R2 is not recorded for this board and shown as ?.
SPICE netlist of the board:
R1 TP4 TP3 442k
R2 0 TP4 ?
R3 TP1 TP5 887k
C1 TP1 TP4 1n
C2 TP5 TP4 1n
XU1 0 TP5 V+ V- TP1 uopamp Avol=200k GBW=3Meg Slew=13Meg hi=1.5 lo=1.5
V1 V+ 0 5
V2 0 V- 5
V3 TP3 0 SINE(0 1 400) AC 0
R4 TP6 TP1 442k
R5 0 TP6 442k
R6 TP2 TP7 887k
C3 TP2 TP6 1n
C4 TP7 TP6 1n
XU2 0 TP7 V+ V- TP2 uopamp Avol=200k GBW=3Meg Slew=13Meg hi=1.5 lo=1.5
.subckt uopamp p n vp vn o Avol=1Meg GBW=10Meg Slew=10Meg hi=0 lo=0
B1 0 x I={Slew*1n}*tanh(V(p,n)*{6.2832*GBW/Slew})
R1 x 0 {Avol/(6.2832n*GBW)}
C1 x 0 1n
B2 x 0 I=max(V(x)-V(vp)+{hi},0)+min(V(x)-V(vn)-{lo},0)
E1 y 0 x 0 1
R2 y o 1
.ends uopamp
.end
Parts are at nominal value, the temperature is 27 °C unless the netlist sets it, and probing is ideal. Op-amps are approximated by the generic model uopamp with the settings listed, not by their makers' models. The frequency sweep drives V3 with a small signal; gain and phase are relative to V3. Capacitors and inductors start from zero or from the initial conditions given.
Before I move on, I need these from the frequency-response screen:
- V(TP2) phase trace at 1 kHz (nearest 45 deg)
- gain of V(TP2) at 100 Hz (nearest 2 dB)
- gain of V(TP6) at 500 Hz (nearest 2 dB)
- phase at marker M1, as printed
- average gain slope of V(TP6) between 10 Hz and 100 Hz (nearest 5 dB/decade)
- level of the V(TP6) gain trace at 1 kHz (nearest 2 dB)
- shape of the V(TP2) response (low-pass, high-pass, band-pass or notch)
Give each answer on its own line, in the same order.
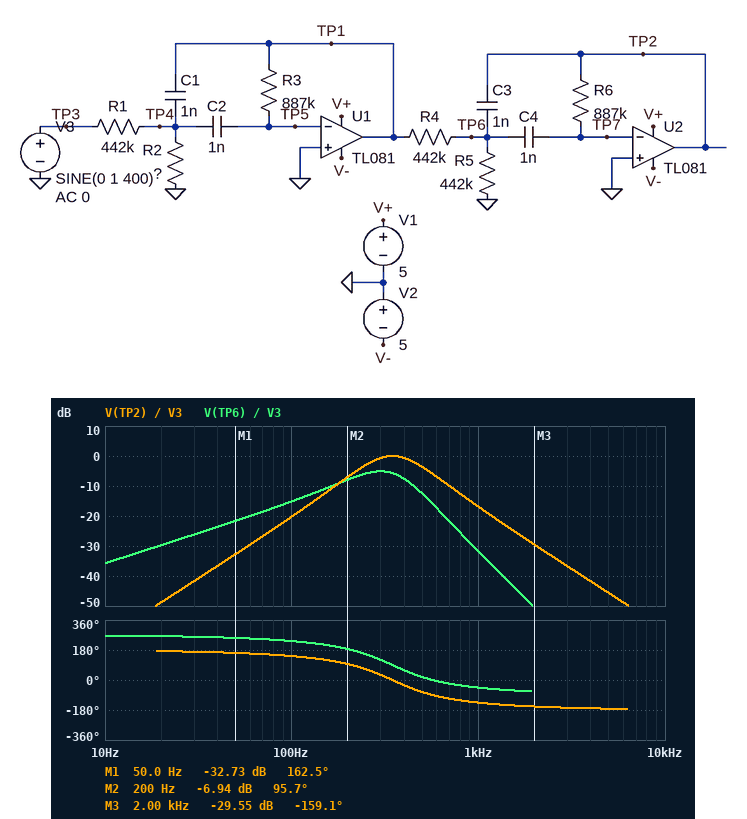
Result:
-135 deg
-20 dB
-12 dB
162.5 deg
20 dB/decade
-32 dB
band-pass
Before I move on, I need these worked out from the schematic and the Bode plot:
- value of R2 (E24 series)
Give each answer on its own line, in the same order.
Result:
620 kΩ
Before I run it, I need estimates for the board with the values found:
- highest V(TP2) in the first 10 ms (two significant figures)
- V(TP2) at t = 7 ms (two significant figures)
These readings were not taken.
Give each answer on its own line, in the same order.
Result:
940 mV
-910 mV
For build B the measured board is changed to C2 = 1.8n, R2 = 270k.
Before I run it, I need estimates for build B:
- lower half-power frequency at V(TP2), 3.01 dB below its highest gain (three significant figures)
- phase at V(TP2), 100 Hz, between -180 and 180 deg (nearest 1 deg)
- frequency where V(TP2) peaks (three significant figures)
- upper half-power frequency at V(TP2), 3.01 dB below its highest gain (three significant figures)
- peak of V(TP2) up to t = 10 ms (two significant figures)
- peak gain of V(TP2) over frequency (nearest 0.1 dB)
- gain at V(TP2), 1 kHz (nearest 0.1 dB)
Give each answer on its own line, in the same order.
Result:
243 Hz
145 deg
330 Hz
451 Hz
1.1 V
2.0 dB
-16.8 dB
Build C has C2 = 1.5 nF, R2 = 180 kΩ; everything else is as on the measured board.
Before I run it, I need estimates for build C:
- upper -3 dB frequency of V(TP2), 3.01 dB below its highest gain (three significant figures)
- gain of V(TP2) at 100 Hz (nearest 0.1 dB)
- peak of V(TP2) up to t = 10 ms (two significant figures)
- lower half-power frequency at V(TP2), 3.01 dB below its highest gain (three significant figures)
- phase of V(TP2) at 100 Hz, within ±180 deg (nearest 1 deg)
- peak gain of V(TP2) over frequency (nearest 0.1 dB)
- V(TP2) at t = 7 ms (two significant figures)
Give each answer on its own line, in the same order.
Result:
495 Hz
-22.7 dB
1.2 V
284 Hz
151 deg
1.6 dB
-1.2 V
